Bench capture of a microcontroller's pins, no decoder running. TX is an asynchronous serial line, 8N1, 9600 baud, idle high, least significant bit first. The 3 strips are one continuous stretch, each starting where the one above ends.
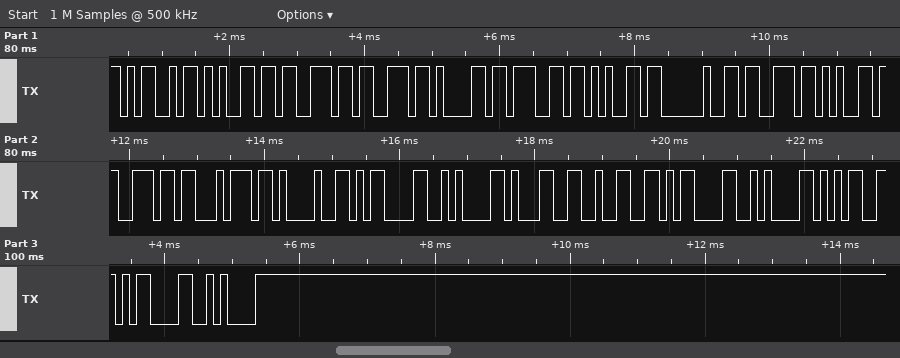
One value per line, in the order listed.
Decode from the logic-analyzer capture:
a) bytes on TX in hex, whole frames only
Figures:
4D 65 73 73 61 67 65 20 73 65 6E 74 21 0D 0A 31 32 0D 0A 35 0D 0A
